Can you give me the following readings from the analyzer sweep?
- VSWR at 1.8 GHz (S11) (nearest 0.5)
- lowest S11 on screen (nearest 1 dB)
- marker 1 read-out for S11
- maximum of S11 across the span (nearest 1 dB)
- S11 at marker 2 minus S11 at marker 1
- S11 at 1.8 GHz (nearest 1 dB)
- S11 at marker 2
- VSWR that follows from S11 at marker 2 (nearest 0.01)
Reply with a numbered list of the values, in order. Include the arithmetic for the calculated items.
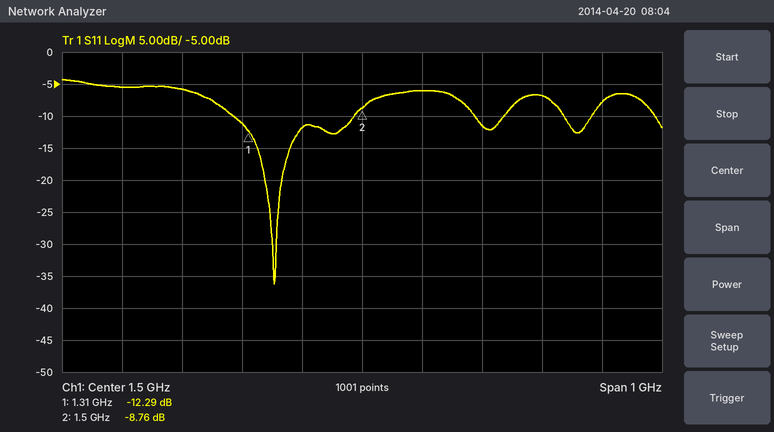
1. |Γ| = 10^(-7/20) = 0.4467; VSWR = (1 + 0.4467)/(1 − 0.4467) ≈ 2.61, so 2.5 to the nearest 0.5
2. -36 dB
3. -12.29 dB
4. -4 dB
5. -8.76 − (-12.29) = 3.53 dB
6. -7 dB
7. -8.76 dB
8. (1 + 0.3648)/(1 − 0.3648) ≈ 2.15
